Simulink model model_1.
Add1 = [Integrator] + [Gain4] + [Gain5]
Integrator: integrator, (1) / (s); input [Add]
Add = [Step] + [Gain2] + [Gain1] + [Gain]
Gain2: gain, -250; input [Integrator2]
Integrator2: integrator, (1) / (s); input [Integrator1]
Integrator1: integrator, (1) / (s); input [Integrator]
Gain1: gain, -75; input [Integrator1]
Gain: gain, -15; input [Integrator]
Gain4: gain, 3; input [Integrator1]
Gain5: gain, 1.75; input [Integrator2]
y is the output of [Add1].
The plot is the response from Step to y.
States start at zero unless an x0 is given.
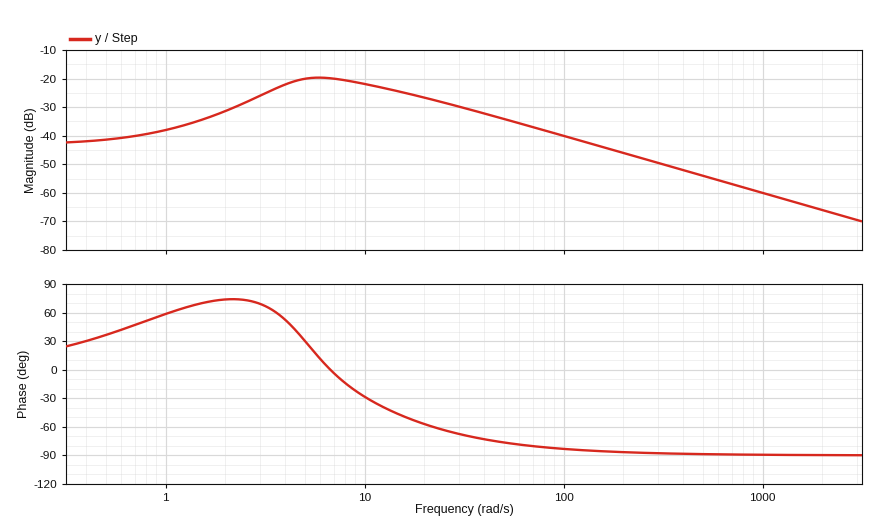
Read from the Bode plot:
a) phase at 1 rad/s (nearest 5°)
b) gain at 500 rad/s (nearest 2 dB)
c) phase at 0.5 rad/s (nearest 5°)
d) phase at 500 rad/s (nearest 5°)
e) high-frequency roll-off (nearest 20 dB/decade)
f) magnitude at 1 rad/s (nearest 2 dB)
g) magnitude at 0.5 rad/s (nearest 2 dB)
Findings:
60°
-54 dB
35°
-90°
-20 dB/decade
-38 dB
-42 dB
